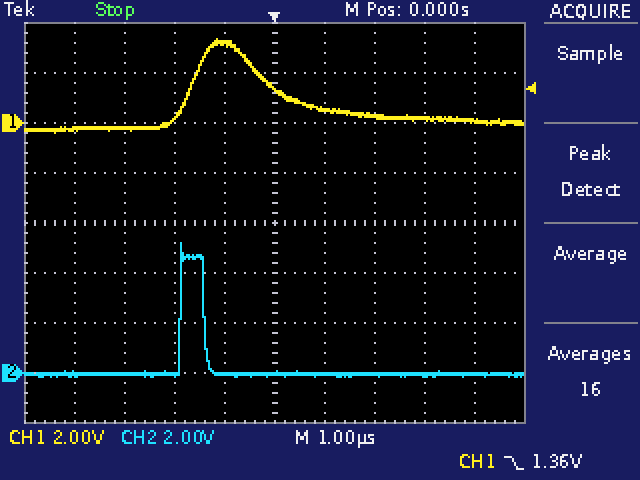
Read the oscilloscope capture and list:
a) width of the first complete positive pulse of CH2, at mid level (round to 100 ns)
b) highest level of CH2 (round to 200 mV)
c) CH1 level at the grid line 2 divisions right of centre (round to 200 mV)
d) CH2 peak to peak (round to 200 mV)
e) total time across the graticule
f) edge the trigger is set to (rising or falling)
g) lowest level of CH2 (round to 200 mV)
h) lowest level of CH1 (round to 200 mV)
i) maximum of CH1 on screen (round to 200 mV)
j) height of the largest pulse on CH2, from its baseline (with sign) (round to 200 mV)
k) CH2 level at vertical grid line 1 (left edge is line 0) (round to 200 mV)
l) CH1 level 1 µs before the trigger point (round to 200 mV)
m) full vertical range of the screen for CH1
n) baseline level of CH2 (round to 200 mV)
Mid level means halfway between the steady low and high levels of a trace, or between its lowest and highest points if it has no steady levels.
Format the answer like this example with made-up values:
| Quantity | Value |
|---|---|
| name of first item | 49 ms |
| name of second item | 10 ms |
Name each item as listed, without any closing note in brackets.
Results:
| Quantity | Value |
|---|---|
| width of the first complete positive pulse of CH2, at mid level | 500 ns |
| highest level of CH2 | 5.2 V |
| CH1 level at the grid line 2 divisions right of centre | 200 mV |
| CH2 peak to peak | 5.4 V |
| total time across the graticule | 10 µs |
| edge the trigger is set to | falling |
| lowest level of CH2 | -200 mV |
| lowest level of CH1 | -400 mV |
| maximum of CH1 on screen | 3.4 V |
| height of the largest pulse on CH2, from its baseline (with sign) | +5.2 V |
| CH2 level at vertical grid line 1 (left edge is line 0) | 0.0 V |
| CH1 level 1 µs before the trigger point | 3.2 V |
| full vertical range of the screen for CH1 | 16 V |
| baseline level of CH2 | 0.0 V |
